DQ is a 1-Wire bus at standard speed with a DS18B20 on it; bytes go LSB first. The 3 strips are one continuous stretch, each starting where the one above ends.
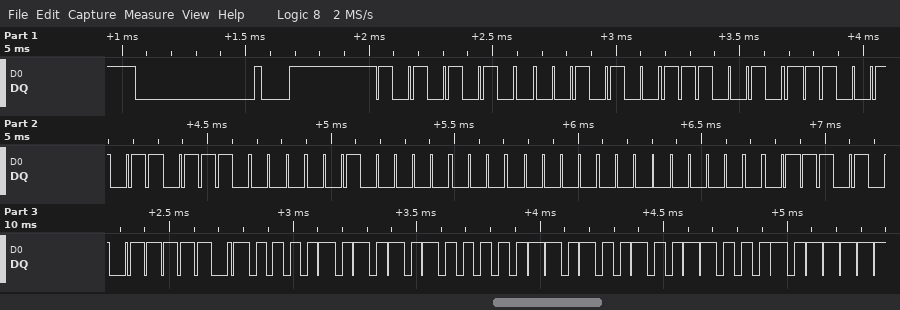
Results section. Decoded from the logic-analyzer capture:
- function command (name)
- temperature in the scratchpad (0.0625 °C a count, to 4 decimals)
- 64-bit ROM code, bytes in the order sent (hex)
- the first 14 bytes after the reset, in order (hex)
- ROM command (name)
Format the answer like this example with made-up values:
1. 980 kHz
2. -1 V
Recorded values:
1. Read Scratchpad
2. 85.0000 °C
3. 28 A7 D3 0E 04 00 00 5C
4. 55 28 A7 D3 0E 04 00 00 5C BE 50 05 4B 46
5. Match ROM
